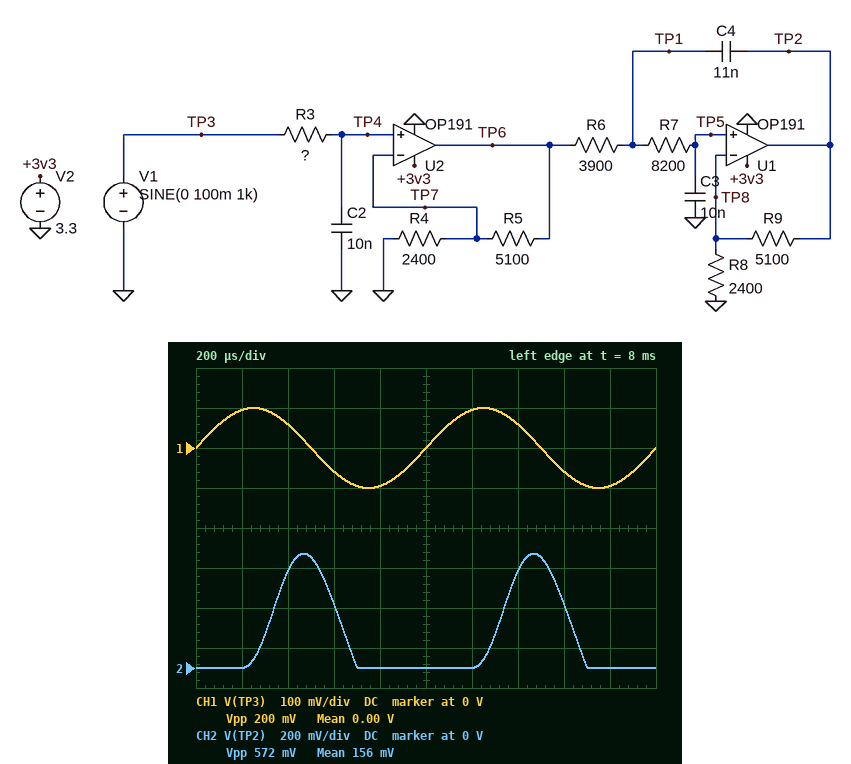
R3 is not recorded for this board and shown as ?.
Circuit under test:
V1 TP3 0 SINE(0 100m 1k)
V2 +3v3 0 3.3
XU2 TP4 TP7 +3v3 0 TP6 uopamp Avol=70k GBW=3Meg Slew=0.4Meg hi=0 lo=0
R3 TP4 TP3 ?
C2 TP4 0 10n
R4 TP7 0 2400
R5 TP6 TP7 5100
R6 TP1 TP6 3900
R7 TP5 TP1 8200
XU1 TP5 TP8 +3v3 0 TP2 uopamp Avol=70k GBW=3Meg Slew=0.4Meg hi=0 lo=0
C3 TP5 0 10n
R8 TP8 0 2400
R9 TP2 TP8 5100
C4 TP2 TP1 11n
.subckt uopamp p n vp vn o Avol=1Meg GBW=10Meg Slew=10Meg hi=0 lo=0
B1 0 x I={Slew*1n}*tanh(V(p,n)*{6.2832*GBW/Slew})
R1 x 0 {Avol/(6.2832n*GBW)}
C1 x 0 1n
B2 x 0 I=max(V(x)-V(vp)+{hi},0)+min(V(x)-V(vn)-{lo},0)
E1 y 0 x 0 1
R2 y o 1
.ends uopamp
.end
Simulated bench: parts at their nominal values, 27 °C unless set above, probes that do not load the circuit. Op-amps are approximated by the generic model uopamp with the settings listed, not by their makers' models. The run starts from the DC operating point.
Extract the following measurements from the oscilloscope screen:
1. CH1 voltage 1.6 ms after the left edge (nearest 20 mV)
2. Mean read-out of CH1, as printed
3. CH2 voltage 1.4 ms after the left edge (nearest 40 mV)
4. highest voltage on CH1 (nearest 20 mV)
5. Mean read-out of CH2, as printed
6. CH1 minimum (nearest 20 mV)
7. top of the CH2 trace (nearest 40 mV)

-60 mV
0.00 V
480 mV
100 mV
156 mV
-100 mV
560 mV
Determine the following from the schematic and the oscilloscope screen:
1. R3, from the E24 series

30 kΩ
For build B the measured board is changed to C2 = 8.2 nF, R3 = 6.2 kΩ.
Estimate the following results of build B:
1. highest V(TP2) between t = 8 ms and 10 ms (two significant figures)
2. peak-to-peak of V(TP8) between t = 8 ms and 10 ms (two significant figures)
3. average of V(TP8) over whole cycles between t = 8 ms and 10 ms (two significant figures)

1.2 V
370 mV
100 mV
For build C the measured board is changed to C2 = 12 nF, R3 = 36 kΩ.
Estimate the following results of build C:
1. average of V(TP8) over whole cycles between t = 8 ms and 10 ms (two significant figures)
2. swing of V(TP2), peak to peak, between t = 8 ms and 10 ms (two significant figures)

37 mV
420 mV
